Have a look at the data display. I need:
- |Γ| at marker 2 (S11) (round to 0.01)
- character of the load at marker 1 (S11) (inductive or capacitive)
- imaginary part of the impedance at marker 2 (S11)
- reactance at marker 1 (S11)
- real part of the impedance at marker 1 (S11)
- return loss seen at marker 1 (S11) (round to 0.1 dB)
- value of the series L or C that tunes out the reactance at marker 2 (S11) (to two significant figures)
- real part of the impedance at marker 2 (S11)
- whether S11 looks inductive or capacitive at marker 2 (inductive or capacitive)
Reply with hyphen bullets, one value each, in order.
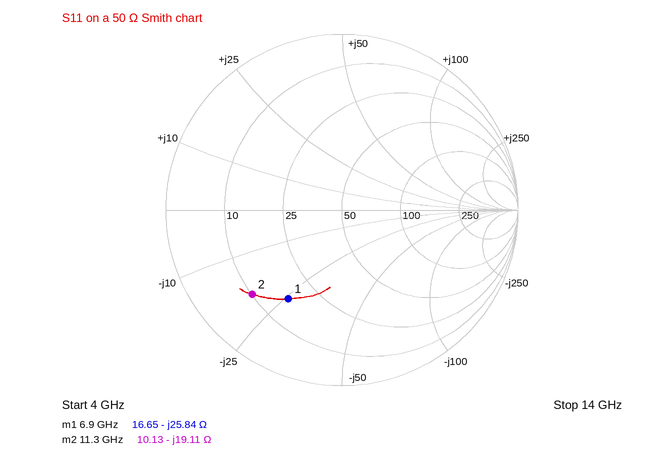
- 0.70
- capacitive
- -19.11 Ω
- -25.84 Ω
- 16.65 Ω
- 4.6 dB
- 270 pH
- 10.13 Ω
- capacitive
